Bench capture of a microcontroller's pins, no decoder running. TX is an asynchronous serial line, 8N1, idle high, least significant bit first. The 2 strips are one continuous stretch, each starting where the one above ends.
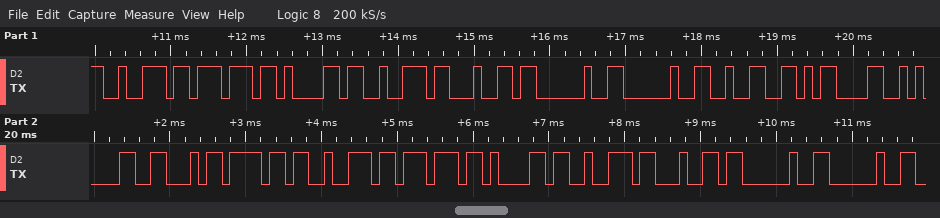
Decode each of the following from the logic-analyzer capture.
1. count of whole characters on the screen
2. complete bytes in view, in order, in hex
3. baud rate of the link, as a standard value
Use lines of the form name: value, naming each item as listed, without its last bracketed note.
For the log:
count of whole characters on the screen: 19
complete bytes in view, in order, in hex: 0x72 0x77 0x61 0x72 0x64 0x20 0x20 0x32 0x0D 0x0A 0x46 0x6F 0x72 0x77 0x61 0x72 0x64 0x20 0x20
baud rate of the link, as a standard value: 9600 baud
